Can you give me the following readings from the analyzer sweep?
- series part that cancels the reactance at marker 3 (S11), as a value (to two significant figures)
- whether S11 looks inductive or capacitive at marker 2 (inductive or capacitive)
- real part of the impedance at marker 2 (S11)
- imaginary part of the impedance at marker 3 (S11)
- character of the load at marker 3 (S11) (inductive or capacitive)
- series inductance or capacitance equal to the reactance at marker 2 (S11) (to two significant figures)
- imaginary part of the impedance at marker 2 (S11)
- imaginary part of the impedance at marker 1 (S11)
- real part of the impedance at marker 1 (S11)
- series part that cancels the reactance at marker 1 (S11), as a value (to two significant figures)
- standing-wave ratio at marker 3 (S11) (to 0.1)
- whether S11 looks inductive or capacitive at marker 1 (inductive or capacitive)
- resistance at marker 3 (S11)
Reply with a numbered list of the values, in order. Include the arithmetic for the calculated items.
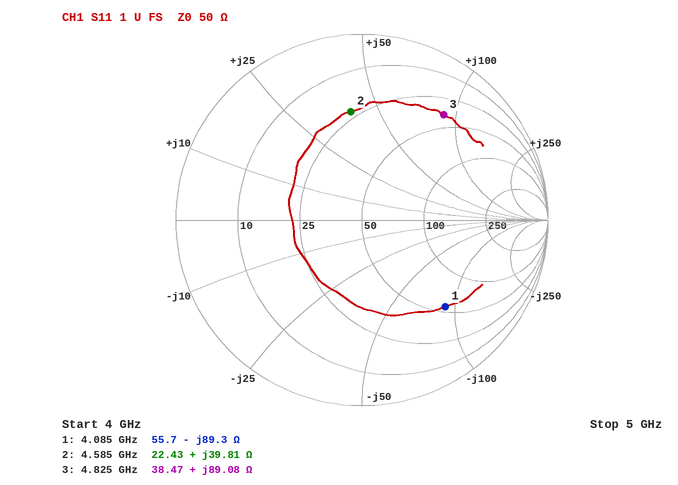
1. C = 1/(2π × 4.825 GHz × 89.08 Ω) ≈ 370 fF
2. inductive
3. 22.43 Ω
4. +89.08 Ω
5. inductive
6. L = 39.81 Ω/(2π × 4.585 GHz) ≈ 1.4 nH
7. +39.81 Ω
8. -89.3 Ω
9. 55.7 Ω
10. L = 89.3 Ω/(2π × 4.085 GHz) ≈ 3.5 nH
11. 6.0
12. capacitive
13. 38.47 Ω
